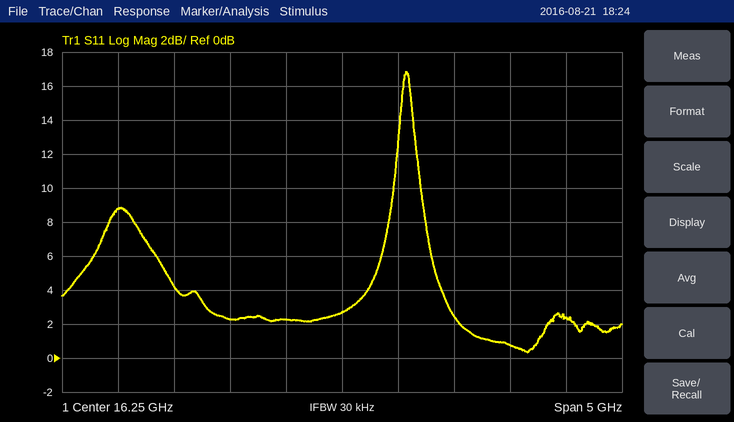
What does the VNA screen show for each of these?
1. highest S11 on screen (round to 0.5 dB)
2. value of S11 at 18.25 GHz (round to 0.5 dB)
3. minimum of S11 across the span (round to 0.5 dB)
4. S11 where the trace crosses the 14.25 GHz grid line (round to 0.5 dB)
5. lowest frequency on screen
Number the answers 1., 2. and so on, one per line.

1. 17.0 dB
2. 2.5 dB
3. 0.5 dB
4. 9.0 dB
5. 13.75 GHz
